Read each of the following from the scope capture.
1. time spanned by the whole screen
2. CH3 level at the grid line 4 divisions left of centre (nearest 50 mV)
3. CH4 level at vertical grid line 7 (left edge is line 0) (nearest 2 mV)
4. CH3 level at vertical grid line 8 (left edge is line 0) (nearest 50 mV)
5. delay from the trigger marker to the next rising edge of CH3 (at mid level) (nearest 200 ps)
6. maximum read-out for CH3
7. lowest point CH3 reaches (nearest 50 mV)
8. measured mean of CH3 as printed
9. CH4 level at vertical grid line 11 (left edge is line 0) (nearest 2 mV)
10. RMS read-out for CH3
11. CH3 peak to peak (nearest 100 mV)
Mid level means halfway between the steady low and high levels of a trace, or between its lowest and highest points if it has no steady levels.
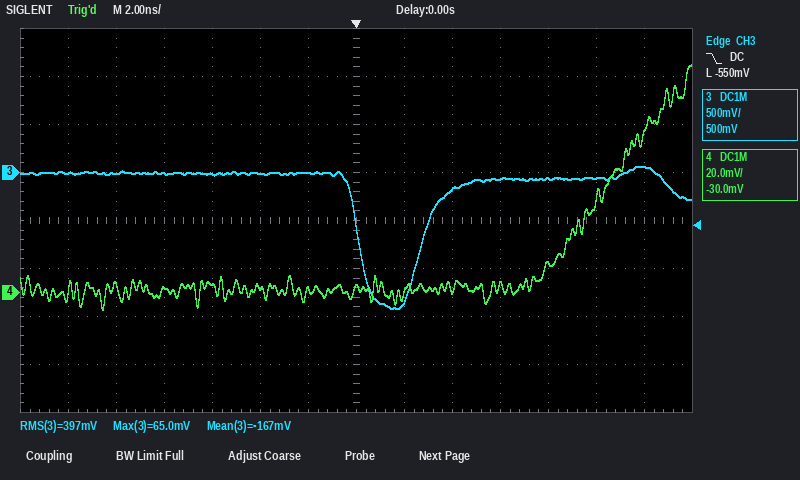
28 ns
0 mV
2 mV
-1.35 V
2.8 ns
65.0 mV
-1.40 V
-167 mV
12 mV
397 mV
1.50 V
